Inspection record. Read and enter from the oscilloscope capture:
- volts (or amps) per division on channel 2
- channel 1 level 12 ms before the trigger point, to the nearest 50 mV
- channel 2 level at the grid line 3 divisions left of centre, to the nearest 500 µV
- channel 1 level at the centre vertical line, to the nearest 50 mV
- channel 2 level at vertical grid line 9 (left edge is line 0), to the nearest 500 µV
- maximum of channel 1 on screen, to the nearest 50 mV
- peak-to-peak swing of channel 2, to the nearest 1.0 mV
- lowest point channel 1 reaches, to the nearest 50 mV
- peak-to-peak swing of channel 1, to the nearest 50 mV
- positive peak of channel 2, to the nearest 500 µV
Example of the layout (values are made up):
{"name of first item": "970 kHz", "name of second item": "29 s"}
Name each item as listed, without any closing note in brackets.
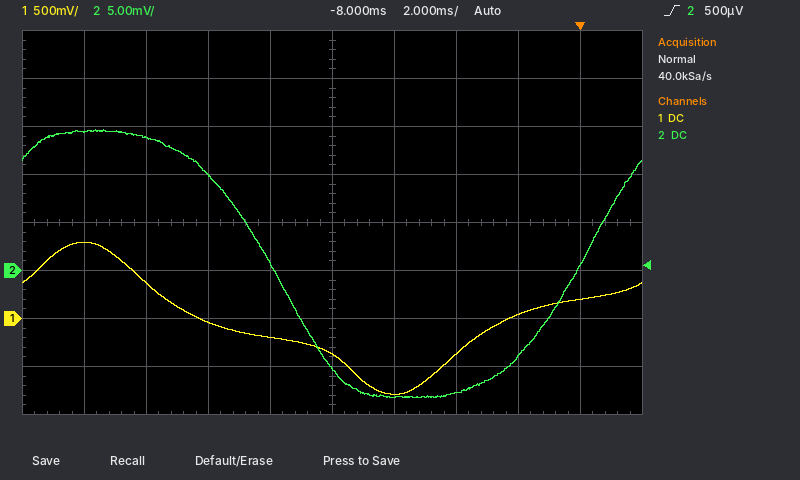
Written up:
{"volts (or amps) per division on channel 2": "5 mV", "channel 1 level 12 ms before the trigger point, to the nearest 50 mV": "-50 mV", "channel 2 level at the grid line 3 divisions left of centre, to the nearest 500 µV": "14.0 mV", "channel 1 level at the centre vertical line, to the nearest 50 mV": "-350 mV", "channel 2 level at vertical grid line 9 (left edge is line 0), to the nearest 500 µV": "500 µV", "maximum of channel 1 on screen, to the nearest 50 mV": "800 mV", "peak-to-peak swing of channel 2, to the nearest 1.0 mV": "28.0 mV", "lowest point channel 1 reaches, to the nearest 50 mV": "-800 mV", "peak-to-peak swing of channel 1, to the nearest 50 mV": "1.60 V", "positive peak of channel 2, to the nearest 500 µV": "14.5 mV"}
